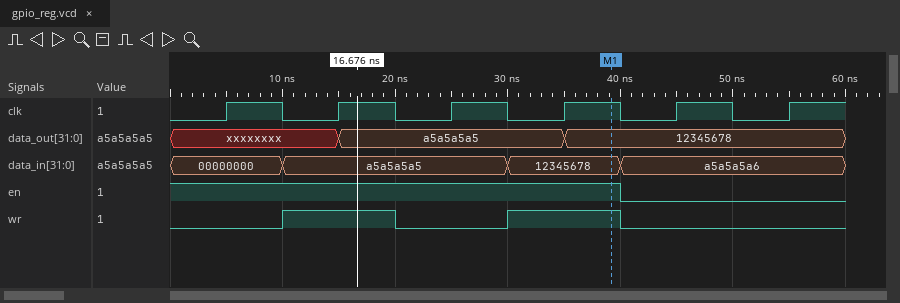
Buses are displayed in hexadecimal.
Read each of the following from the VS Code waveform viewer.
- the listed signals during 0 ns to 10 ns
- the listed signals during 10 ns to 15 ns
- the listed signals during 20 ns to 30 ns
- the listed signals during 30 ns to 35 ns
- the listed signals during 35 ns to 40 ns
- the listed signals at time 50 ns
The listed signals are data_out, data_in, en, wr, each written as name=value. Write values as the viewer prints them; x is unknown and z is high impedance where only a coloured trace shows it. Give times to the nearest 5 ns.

data_out=xxxxxxxx, data_in=00000000, en=1, wr=0
data_out=xxxxxxxx, data_in=a5a5a5a5, en=1, wr=1
data_out=a5a5a5a5, data_in=a5a5a5a5, en=1, wr=0
data_out=a5a5a5a5, data_in=12345678, en=1, wr=1
data_out=12345678, data_in=12345678, en=1, wr=1
data_out=12345678, data_in=a5a5a5a6, en=0, wr=0
